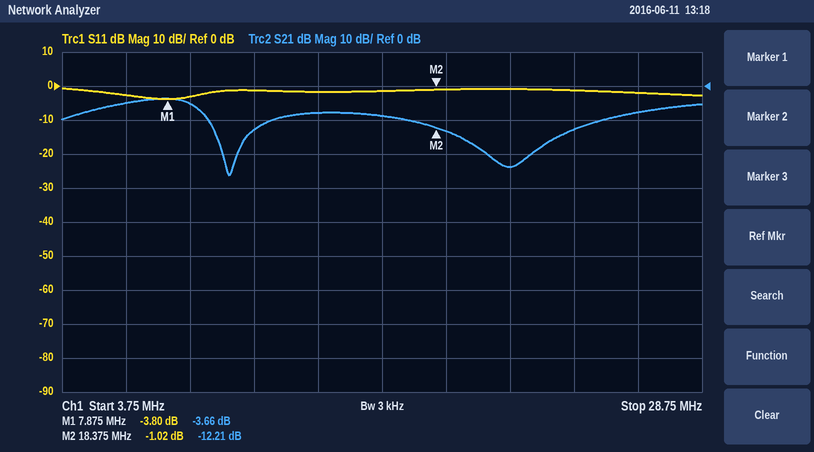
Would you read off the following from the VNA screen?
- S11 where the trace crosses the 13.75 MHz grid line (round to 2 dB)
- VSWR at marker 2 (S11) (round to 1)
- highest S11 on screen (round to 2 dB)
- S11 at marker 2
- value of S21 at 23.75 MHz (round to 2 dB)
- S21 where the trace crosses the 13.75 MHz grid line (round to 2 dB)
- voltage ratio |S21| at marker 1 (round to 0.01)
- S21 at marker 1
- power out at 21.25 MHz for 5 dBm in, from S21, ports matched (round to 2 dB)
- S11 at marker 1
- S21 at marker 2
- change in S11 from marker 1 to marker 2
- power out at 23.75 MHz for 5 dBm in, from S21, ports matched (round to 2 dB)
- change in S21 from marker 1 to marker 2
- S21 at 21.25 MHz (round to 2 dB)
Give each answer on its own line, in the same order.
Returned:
-2 dB
17
0 dB
-1.02 dB
-12 dB
-8 dB
0.66
-3.66 dB
-18 dBm
-3.80 dB
-12.21 dB
2.78 dB
-8 dBm
-8.55 dB
-24 dB
